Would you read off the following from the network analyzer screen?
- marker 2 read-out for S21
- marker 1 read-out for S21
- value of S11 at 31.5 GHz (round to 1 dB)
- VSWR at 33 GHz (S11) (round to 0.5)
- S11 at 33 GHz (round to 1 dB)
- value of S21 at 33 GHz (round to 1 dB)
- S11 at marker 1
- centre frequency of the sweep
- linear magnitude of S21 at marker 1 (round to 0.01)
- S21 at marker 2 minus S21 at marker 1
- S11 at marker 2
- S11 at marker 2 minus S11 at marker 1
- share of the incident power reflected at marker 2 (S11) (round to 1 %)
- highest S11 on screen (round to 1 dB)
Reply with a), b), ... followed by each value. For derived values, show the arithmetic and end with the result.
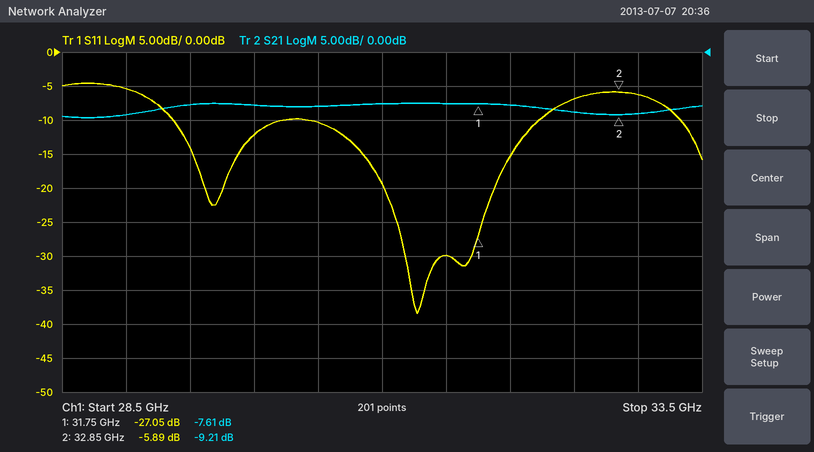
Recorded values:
a) -9.21 dB
b) -7.61 dB
c) -30 dB
d) |Γ| = 10^(-6/20) = 0.5012; VSWR = (1 + 0.5012)/(1 − 0.5012) ≈ 3.0
e) -6 dB
f) -9 dB
g) -27.05 dB
h) 31 GHz
i) 10^(-7.61/20) ≈ 0.42
j) -9.21 − (-7.61) = -1.60 dB
k) -5.89 dB
l) -5.89 − (-27.05) = 21.16 dB
m) 10^(-5.89/10) ≈ 26 %
n) -5 dB
